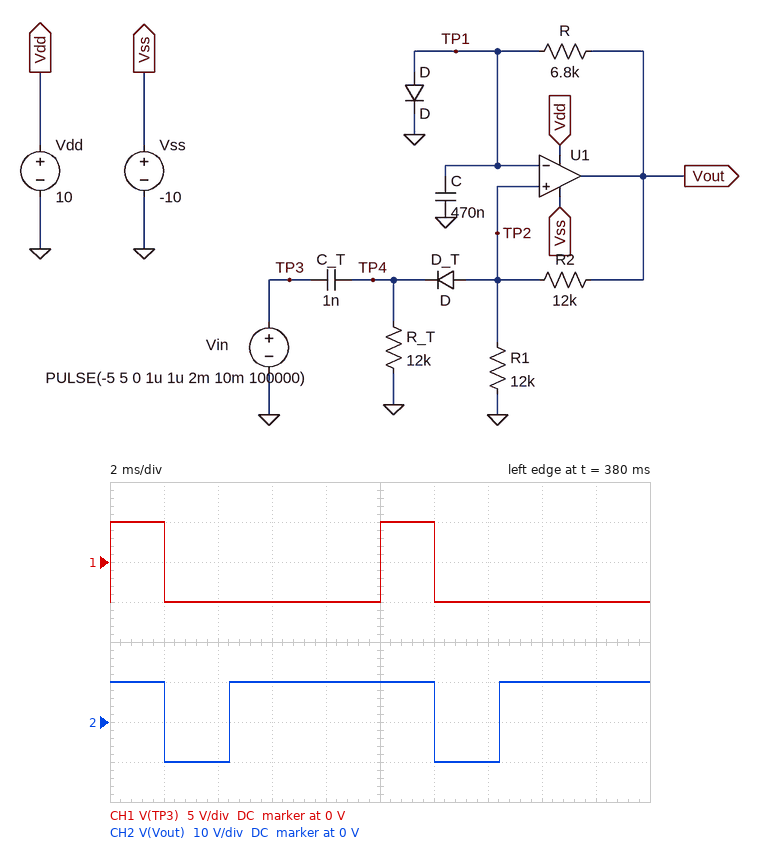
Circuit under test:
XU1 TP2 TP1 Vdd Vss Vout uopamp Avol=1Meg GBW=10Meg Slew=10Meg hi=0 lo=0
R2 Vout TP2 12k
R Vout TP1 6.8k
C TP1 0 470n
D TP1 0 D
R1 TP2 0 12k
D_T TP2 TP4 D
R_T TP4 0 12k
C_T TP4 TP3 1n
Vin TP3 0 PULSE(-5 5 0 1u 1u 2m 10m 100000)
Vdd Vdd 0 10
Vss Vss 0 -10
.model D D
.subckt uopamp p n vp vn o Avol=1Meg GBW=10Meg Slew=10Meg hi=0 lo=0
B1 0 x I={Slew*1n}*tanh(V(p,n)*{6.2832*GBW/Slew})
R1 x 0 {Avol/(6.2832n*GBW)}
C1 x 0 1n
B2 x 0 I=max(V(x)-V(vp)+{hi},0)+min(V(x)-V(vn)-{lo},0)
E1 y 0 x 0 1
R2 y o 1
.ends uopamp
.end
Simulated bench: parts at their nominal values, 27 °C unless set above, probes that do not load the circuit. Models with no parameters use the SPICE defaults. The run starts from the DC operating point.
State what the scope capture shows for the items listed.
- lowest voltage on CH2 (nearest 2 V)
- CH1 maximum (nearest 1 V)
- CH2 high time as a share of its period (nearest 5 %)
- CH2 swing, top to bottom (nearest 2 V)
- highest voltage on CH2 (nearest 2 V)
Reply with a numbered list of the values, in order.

1. -10 V
2. 5 V
3. 75 %
4. 20 V
5. 10 V
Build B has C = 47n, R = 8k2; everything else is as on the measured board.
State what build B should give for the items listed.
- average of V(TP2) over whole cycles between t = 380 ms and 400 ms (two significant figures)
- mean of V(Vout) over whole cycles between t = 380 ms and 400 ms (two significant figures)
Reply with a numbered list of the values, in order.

1. 3.3 V
2. 9.4 V
